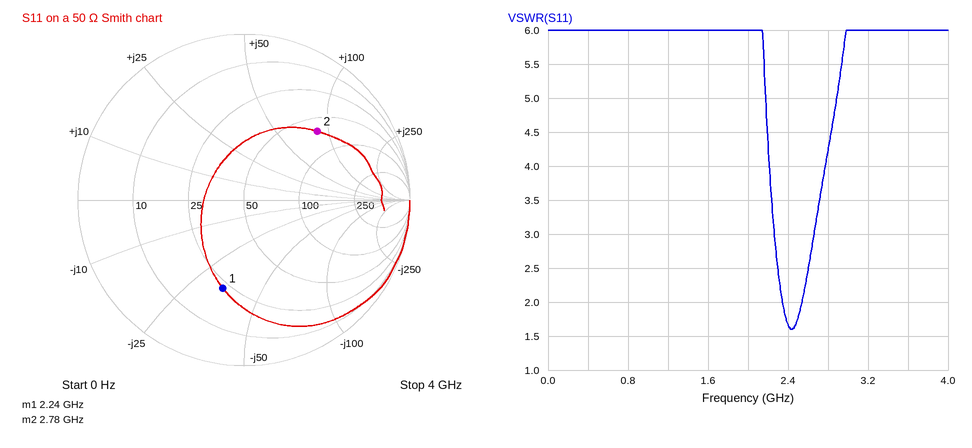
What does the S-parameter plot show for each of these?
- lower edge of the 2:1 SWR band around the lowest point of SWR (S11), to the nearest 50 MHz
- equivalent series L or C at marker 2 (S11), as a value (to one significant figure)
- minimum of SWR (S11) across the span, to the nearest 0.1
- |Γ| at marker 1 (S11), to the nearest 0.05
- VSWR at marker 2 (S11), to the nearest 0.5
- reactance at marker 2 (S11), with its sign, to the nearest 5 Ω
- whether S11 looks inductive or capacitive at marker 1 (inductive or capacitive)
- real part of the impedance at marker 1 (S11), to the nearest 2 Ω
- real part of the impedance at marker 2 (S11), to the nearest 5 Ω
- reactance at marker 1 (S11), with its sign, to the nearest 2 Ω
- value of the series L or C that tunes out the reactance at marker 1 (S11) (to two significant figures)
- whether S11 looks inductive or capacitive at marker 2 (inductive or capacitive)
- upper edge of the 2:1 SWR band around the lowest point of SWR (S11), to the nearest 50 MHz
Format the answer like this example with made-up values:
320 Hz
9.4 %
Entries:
2.35 GHz
5 nH
1.6
0.55
4.0
+85 Ω
capacitive
22 Ω
65 Ω
-34 Ω
2.4 nH
inductive
2.55 GHz
